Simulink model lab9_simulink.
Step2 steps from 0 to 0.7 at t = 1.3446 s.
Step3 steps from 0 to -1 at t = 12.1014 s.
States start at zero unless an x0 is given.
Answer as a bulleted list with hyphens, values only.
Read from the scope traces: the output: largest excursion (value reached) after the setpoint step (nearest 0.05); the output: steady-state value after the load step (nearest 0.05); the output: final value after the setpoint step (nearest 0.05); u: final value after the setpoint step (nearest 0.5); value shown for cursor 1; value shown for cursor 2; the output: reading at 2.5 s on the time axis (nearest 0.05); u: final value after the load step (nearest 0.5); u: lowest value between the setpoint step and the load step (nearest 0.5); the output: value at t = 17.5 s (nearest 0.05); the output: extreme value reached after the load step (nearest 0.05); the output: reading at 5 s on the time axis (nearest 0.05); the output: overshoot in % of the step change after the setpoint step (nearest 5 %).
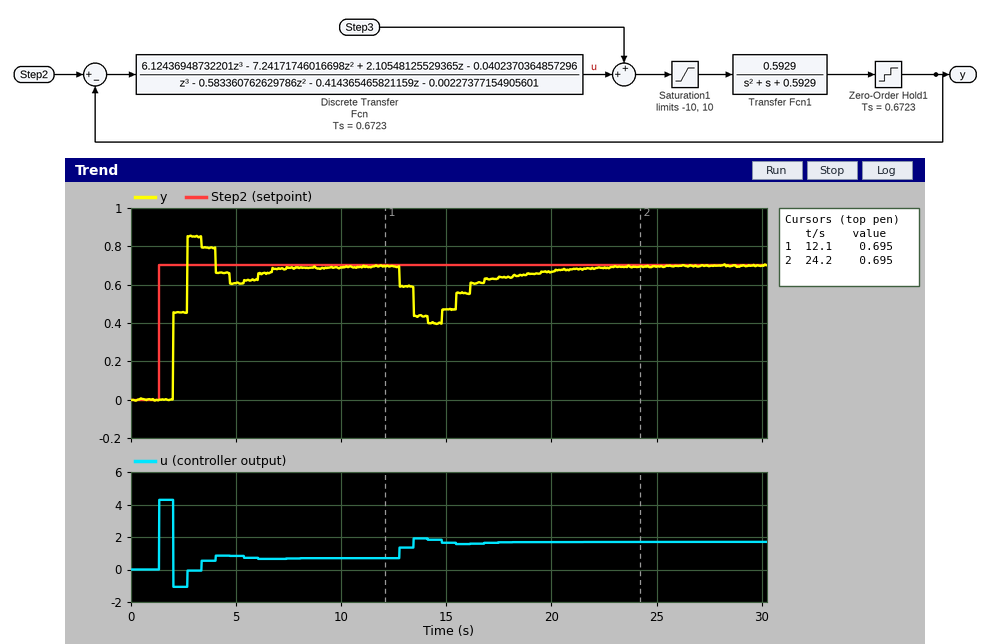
- 0.85
- 0.70
- 0.70
- 0.5
- 0.695
- 0.695
- 0.45
- 1.5
- -1.0
- 0.65
- 0.40
- 0.60
- 20 %
